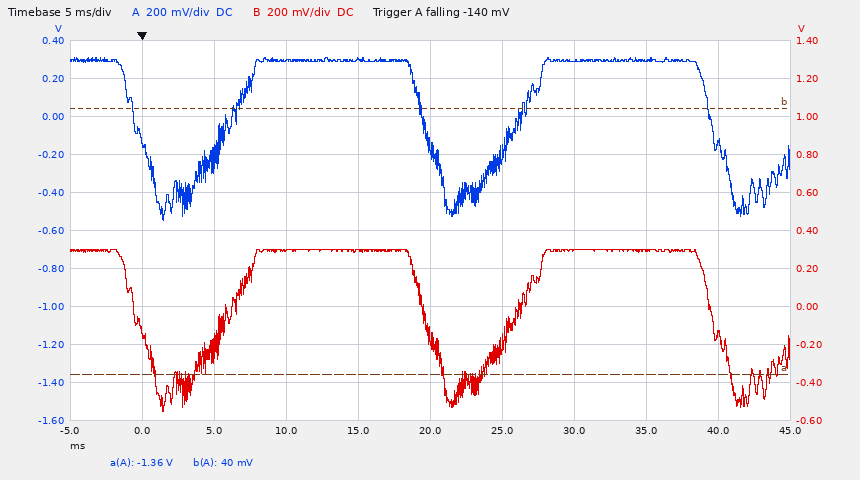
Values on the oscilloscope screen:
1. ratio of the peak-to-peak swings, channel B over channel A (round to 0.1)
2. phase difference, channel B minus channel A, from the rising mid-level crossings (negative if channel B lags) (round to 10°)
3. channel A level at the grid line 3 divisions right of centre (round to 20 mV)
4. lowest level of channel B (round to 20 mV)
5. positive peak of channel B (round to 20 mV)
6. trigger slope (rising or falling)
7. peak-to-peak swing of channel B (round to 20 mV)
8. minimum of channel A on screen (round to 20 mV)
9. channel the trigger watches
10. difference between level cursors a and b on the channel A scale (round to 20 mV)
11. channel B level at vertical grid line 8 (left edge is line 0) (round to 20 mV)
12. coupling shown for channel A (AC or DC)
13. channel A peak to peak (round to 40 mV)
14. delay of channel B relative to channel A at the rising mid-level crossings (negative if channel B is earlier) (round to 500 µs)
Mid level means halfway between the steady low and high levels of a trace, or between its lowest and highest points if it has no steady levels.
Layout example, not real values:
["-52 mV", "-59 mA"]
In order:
["1.0", "0°", "300 mV", "-560 mV", "300 mV", "falling", "860 mV", "-540 mV", "channel A", "1.40 V", "300 mV", "DC", "840 mV", "0.0 ms"]
